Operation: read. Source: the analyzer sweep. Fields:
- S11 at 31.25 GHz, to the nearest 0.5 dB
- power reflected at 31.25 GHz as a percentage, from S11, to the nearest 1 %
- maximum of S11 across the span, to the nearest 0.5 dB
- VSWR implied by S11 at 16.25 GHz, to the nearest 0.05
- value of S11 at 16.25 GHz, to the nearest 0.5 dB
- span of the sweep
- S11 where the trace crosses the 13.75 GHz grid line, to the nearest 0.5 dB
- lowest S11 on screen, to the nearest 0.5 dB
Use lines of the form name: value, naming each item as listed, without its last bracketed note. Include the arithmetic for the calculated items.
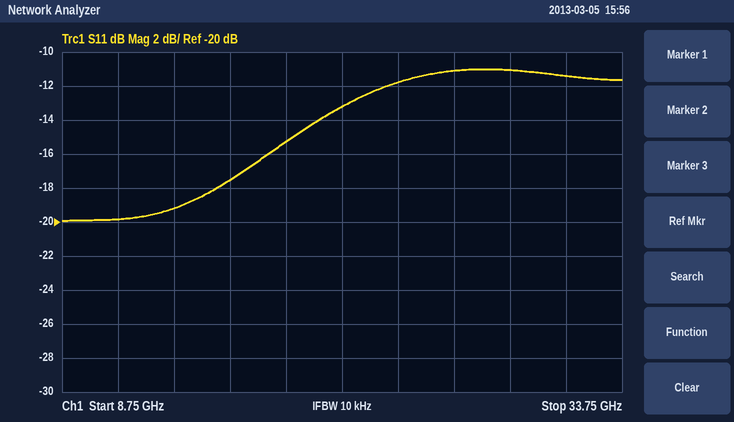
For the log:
S11 at 31.25 GHz, to the nearest 0.5 dB: -11.5 dB
power reflected at 31.25 GHz as a percentage, from S11, to the nearest 1 %: 10^(-11.5/10) ≈ 7 %
maximum of S11 across the span, to the nearest 0.5 dB: -11.0 dB
VSWR implied by S11 at 16.25 GHz, to the nearest 0.05: |Γ| = 10^(-17.5/20) = 0.1334; VSWR = (1 + 0.1334)/(1 − 0.1334) ≈ 1.31, so 1.30 to the nearest 0.05
value of S11 at 16.25 GHz, to the nearest 0.5 dB: -17.5 dB
span of the sweep: 25 GHz
S11 where the trace crosses the 13.75 GHz grid line, to the nearest 0.5 dB: -19.0 dB
lowest S11 on screen, to the nearest 0.5 dB: -20.0 dB
